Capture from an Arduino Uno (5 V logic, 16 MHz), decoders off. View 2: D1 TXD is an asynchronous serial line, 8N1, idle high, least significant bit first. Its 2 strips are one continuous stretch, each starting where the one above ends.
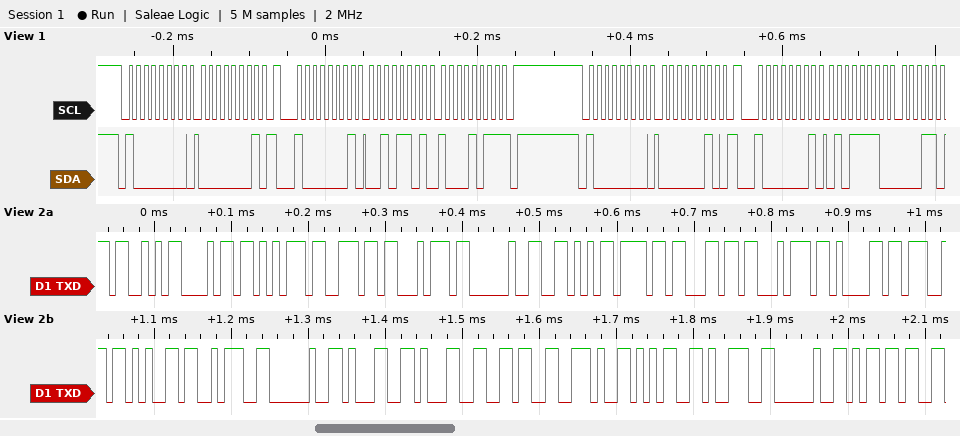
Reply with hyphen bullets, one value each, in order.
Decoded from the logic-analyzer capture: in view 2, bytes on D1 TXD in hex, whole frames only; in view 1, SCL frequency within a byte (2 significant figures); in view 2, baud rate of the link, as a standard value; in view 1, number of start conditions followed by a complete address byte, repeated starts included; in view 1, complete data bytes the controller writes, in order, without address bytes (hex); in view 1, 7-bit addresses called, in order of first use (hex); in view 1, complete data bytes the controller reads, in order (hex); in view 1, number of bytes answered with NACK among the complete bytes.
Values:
- 53 68 75 6E 74 20 56 6F 6C 74 61 67 65 3A 20 31 31 36 2E 35 39 20 6D
- 100 kHz
- 115200 baud
- 4
- 01 02
- 0x40
- 2D 8B 5E
- 1
